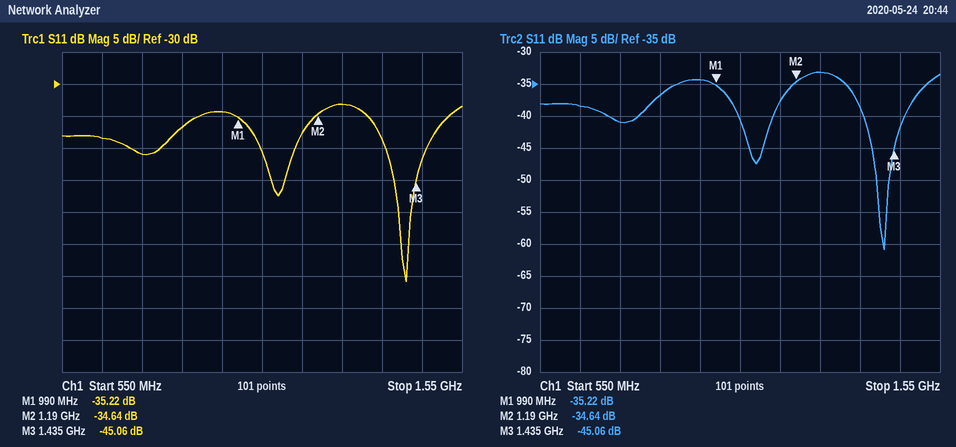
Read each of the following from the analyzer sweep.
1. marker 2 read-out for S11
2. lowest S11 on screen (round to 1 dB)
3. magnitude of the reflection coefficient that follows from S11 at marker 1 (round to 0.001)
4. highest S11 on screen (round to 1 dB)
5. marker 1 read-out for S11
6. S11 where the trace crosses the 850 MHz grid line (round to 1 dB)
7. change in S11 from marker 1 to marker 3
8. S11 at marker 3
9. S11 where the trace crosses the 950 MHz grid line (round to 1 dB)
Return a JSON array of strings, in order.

["-34.64 dB", "-61 dB", "0.017", "-33 dB", "-35.22 dB", "-37 dB", "-9.84 dB", "-45.06 dB", "-34 dB"]
